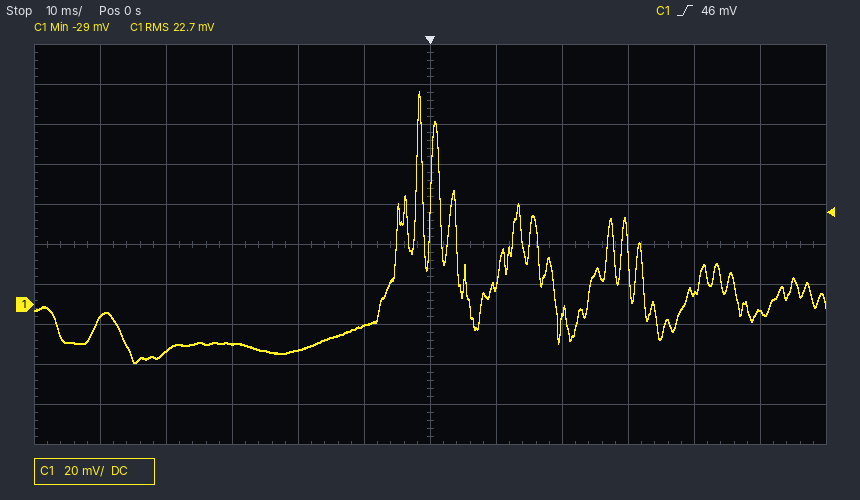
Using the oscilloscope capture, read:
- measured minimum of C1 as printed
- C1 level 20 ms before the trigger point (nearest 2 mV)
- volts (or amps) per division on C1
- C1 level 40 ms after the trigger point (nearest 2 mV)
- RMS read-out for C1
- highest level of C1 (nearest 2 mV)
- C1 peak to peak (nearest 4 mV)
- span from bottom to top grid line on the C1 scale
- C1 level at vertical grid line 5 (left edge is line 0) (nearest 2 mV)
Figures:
-29 mV
-22 mV
20 mV
6 mV
22.7 mV
106 mV
136 mV
200 mV
-10 mV
